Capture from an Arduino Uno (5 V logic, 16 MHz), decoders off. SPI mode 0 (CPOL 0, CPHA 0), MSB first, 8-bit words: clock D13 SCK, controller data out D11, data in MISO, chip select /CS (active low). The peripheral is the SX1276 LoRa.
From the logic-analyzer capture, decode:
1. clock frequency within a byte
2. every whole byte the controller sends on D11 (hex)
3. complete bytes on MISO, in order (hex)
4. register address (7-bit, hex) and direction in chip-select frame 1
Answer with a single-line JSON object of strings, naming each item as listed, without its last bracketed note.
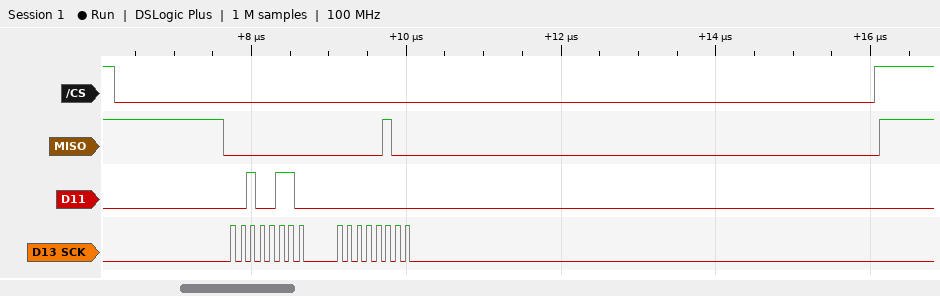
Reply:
{"clock frequency within a byte": "8 MHz", "every whole byte the controller sends on D11": "26 00", "complete bytes on MISO, in order": "00 04", "register address (7-bit, hex) and direction in chip-select frame 1": "0x26 read"}
